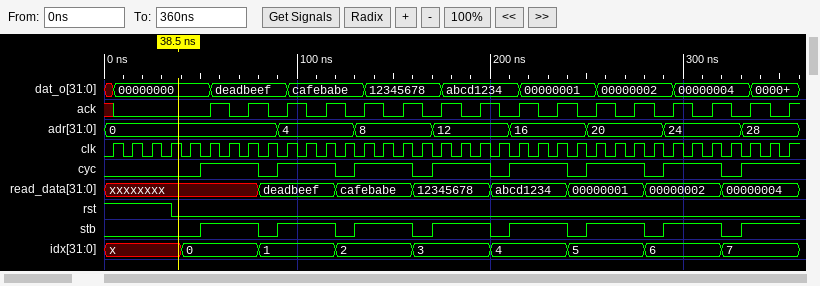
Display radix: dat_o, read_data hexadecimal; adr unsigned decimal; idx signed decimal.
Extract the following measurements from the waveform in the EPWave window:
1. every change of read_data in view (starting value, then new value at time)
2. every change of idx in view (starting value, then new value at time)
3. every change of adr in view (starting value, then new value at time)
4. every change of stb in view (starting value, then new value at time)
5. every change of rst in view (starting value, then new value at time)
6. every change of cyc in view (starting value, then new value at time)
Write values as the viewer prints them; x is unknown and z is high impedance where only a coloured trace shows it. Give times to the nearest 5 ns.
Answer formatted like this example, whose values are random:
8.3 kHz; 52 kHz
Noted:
xxxxxxxx, deadbeef at 80 ns, cafebabe at 120 ns, 12345678 at 160 ns, abcd1234 at 200 ns, 00000001 at 240 ns, 00000002 at 280 ns, 00000004 at 320 ns; x, 0 at 40 ns, 1 at 80 ns, 2 at 120 ns, 3 at 160 ns, 4 at 200 ns, 5 at 240 ns, 6 at 280 ns, 7 at 320 ns; 0, 4 at 90 ns, 8 at 130 ns, 12 at 170 ns, 16 at 210 ns, 20 at 250 ns, 24 at 290 ns, 28 at 330 ns; 0, 1 at 50 ns, 0 at 80 ns, 1 at 90 ns, 0 at 120 ns, 1 at 130 ns, 0 at 160 ns, 1 at 170 ns, 0 at 200 ns, 1 at 210 ns, 0 at 240 ns, 1 at 250 ns, 0 at 280 ns, 1 at 290 ns, 0 at 320 ns, 1 at 330 ns; 1, 0 at 35 ns; 0, 1 at 50 ns, 0 at 80 ns, 1 at 90 ns, 0 at 120 ns, 1 at 130 ns, 0 at 160 ns, 1 at 170 ns, 0 at 200 ns, 1 at 210 ns, 0 at 240 ns, 1 at 250 ns, 0 at 280 ns, 1 at 290 ns, 0 at 320 ns, 1 at 330 ns
